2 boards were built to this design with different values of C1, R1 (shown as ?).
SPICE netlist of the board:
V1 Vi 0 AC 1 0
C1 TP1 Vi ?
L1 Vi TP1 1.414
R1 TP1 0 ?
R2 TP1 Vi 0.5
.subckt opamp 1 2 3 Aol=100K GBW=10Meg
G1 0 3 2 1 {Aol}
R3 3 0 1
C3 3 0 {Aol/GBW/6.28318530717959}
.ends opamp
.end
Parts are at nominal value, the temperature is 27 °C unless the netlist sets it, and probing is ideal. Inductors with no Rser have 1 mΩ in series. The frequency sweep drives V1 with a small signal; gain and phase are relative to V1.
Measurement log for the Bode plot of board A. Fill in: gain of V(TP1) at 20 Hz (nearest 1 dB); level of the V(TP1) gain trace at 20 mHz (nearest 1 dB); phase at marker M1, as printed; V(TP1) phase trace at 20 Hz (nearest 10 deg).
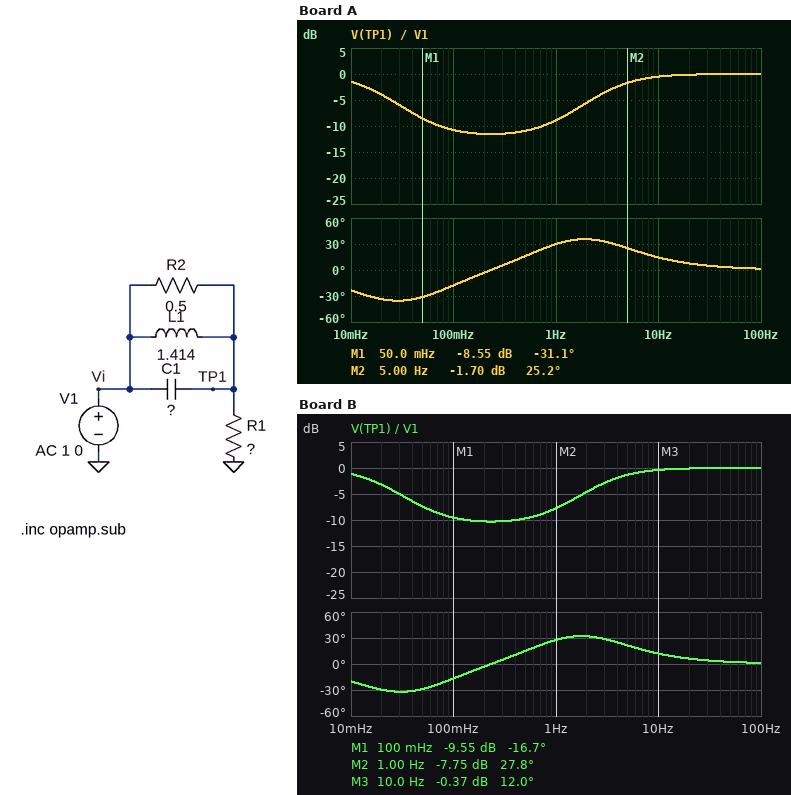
0 dB
-4 dB
-31.1 deg
10 deg
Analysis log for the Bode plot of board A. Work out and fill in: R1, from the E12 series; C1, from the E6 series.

0.18 Ω
330 mF
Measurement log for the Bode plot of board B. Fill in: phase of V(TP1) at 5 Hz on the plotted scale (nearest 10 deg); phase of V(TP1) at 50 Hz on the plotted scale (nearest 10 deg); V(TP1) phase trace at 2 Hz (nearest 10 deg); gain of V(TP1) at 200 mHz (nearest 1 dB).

20 deg
0 deg
30 deg
-10 dB
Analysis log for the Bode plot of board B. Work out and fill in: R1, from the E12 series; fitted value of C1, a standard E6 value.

0.22 Ω
330 mF
